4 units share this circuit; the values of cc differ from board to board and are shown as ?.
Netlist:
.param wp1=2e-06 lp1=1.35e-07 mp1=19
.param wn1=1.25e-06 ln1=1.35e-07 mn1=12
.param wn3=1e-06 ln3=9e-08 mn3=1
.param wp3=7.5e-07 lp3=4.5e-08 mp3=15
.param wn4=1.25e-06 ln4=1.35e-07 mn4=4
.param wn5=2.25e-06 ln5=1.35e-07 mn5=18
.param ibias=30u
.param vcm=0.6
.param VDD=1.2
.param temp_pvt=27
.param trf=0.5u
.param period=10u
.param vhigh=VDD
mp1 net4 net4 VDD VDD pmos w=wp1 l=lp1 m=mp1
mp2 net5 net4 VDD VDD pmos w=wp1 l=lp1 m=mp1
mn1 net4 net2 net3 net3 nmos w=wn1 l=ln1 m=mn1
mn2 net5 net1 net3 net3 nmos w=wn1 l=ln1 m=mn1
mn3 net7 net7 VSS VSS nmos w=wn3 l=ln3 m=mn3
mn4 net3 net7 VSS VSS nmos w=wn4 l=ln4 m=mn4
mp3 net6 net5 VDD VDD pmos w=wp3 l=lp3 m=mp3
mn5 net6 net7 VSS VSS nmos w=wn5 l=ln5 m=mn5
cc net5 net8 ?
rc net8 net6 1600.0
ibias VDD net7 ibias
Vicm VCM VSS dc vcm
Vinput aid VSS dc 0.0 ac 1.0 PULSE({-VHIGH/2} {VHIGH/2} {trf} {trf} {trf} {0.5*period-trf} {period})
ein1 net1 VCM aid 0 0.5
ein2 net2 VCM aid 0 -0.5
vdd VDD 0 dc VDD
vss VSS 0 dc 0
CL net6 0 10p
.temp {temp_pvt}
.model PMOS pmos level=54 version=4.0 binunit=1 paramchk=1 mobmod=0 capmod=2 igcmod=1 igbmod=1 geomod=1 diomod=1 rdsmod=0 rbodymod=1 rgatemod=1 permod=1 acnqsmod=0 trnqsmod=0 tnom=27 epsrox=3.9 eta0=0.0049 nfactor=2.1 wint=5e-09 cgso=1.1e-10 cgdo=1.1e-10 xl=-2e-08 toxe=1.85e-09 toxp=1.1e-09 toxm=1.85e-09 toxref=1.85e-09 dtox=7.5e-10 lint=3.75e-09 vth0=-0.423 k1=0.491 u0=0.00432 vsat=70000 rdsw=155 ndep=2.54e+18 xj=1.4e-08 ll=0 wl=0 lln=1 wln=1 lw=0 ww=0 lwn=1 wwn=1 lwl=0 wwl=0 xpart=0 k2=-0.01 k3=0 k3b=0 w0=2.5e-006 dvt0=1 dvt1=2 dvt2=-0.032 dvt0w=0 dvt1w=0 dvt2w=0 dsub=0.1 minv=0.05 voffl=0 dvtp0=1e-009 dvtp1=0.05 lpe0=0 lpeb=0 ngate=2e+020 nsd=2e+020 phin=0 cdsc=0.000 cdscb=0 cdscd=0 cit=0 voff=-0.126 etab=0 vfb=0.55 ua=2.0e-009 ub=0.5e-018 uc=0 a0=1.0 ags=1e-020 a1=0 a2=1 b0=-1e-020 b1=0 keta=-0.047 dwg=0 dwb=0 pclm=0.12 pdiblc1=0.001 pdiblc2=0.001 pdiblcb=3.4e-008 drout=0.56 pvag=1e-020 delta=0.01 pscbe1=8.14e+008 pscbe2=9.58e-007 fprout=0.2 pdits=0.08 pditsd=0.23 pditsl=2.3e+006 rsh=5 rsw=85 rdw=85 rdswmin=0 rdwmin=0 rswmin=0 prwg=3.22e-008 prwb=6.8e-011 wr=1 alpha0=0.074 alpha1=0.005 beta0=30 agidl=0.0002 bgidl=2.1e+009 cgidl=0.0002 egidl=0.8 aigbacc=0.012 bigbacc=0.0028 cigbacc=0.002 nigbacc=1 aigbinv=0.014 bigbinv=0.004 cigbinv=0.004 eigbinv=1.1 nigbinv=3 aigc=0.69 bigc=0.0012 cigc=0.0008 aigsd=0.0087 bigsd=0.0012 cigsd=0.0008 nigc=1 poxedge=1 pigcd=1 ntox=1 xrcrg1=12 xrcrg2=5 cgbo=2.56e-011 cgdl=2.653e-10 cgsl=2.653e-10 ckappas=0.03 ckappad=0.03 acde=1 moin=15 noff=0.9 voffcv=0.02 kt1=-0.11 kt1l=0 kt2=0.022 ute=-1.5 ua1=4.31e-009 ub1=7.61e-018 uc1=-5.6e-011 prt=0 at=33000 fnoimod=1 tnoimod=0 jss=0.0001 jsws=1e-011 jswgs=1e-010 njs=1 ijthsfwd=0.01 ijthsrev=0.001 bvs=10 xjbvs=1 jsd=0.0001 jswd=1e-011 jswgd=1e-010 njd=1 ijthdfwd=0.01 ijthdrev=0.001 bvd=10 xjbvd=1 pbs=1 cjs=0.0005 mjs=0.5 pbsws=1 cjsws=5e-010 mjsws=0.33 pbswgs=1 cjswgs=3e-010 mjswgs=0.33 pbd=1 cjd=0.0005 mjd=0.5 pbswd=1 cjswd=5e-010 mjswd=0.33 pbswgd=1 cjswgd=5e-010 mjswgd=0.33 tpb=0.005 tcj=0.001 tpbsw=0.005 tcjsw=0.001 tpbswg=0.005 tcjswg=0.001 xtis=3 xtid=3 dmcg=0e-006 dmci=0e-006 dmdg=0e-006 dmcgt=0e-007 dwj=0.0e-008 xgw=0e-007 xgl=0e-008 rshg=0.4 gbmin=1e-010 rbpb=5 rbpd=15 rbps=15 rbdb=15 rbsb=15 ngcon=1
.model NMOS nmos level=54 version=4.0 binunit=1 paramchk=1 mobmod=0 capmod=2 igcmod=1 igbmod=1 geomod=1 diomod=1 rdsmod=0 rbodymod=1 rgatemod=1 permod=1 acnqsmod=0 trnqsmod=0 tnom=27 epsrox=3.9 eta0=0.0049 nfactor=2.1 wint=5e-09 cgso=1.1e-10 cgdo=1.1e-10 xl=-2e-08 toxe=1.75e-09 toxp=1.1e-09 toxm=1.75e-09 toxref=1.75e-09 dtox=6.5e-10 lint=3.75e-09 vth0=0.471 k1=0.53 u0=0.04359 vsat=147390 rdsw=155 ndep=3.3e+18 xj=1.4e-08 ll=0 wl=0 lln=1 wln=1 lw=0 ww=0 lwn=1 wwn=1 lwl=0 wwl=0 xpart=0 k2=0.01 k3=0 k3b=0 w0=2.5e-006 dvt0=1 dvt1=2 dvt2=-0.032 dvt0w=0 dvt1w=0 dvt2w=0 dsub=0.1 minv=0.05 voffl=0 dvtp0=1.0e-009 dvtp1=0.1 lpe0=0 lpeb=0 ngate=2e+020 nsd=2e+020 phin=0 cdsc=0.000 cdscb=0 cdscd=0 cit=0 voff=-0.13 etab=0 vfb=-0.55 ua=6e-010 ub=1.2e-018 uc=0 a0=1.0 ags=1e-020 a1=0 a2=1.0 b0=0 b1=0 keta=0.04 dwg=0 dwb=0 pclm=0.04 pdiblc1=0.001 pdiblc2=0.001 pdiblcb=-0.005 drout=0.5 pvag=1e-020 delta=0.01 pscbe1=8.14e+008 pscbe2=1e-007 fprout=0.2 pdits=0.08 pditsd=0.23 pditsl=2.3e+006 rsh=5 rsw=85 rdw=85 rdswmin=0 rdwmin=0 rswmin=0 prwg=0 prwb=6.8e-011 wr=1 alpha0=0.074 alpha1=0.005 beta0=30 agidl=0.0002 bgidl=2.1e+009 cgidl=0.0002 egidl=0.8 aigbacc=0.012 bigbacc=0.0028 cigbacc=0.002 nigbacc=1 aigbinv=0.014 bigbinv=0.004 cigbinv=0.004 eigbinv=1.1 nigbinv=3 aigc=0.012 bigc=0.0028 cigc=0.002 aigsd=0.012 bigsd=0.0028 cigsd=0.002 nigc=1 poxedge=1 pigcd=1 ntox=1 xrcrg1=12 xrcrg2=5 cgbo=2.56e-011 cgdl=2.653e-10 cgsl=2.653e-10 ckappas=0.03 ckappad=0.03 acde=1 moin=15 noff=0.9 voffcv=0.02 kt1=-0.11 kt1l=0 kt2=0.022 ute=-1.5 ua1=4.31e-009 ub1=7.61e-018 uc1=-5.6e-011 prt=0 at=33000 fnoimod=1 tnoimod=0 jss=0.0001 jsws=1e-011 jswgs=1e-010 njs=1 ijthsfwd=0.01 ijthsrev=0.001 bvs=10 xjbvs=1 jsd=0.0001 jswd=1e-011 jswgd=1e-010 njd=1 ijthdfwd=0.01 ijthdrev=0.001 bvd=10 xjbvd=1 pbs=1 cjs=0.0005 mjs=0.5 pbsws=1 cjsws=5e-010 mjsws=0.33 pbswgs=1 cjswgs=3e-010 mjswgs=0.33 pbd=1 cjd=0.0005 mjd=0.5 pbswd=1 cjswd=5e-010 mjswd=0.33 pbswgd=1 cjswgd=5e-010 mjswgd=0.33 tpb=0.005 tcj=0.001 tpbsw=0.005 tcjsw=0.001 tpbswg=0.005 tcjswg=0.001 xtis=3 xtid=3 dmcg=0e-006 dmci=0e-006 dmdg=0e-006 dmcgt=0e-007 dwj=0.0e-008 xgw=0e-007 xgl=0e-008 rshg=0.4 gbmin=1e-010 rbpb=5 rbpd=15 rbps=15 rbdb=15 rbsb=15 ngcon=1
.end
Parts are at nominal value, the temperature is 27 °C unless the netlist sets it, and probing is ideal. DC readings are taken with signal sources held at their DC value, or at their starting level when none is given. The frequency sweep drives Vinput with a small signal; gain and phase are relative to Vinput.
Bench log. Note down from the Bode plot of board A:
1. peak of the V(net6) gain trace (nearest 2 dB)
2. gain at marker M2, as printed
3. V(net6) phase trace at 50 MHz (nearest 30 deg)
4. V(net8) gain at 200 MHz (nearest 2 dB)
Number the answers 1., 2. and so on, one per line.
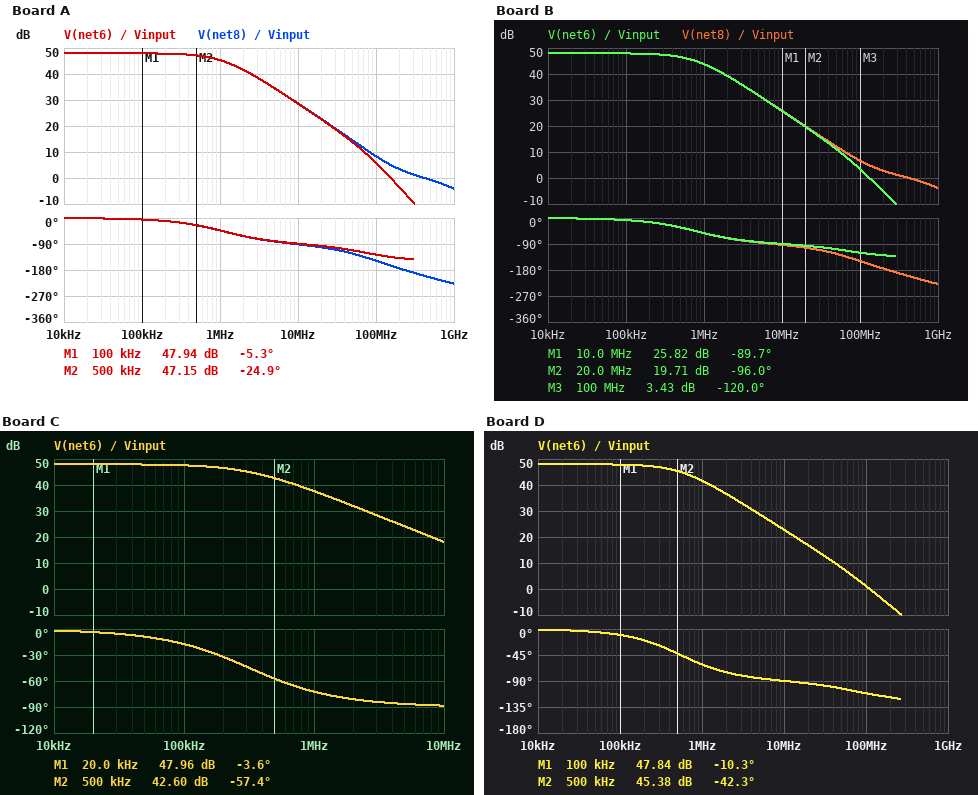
1. 48 dB
2. 47.15 dB
3. -120 deg
4. 4 dB
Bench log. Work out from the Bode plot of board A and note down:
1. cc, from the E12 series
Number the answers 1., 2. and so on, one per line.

1. 330 fF
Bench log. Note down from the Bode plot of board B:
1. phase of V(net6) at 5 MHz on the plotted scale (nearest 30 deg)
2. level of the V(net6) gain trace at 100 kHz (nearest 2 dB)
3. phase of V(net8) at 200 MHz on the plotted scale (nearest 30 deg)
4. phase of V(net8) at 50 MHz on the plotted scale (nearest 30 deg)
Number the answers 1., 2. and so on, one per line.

1. -90 deg
2. 48 dB
3. -180 deg
4. -120 deg
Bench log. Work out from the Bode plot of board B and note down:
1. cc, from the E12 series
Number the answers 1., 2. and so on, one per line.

1. 470 fF
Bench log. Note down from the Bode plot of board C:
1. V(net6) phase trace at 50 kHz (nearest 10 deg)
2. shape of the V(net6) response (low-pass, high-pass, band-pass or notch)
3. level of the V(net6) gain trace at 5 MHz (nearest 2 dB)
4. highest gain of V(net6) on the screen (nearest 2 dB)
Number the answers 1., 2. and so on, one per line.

1. -10 deg
2. low-pass
3. 24 dB
4. 48 dB
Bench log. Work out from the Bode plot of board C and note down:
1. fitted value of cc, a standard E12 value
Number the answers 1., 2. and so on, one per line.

1. 1.2 pF
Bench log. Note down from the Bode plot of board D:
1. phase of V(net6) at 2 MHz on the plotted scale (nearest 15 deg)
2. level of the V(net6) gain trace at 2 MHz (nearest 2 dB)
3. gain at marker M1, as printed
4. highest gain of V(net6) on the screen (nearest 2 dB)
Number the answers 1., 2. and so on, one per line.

1. -75 deg
2. 36 dB
3. 47.84 dB
4. 48 dB
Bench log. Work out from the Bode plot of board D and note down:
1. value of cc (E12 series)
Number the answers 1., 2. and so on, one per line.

1. 680 fF
